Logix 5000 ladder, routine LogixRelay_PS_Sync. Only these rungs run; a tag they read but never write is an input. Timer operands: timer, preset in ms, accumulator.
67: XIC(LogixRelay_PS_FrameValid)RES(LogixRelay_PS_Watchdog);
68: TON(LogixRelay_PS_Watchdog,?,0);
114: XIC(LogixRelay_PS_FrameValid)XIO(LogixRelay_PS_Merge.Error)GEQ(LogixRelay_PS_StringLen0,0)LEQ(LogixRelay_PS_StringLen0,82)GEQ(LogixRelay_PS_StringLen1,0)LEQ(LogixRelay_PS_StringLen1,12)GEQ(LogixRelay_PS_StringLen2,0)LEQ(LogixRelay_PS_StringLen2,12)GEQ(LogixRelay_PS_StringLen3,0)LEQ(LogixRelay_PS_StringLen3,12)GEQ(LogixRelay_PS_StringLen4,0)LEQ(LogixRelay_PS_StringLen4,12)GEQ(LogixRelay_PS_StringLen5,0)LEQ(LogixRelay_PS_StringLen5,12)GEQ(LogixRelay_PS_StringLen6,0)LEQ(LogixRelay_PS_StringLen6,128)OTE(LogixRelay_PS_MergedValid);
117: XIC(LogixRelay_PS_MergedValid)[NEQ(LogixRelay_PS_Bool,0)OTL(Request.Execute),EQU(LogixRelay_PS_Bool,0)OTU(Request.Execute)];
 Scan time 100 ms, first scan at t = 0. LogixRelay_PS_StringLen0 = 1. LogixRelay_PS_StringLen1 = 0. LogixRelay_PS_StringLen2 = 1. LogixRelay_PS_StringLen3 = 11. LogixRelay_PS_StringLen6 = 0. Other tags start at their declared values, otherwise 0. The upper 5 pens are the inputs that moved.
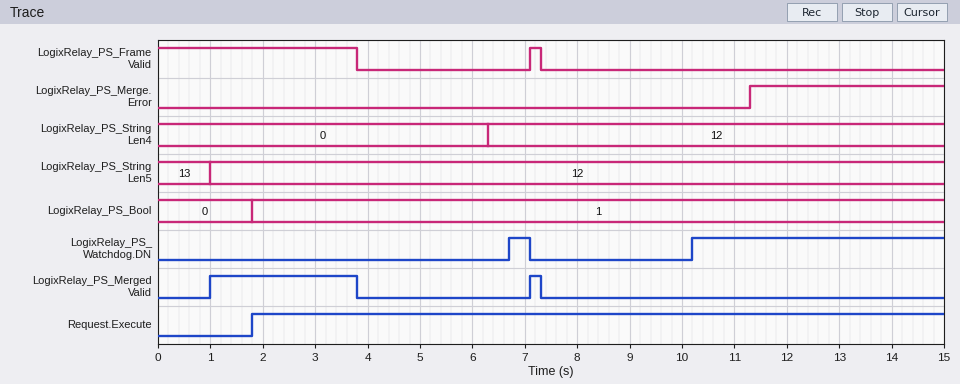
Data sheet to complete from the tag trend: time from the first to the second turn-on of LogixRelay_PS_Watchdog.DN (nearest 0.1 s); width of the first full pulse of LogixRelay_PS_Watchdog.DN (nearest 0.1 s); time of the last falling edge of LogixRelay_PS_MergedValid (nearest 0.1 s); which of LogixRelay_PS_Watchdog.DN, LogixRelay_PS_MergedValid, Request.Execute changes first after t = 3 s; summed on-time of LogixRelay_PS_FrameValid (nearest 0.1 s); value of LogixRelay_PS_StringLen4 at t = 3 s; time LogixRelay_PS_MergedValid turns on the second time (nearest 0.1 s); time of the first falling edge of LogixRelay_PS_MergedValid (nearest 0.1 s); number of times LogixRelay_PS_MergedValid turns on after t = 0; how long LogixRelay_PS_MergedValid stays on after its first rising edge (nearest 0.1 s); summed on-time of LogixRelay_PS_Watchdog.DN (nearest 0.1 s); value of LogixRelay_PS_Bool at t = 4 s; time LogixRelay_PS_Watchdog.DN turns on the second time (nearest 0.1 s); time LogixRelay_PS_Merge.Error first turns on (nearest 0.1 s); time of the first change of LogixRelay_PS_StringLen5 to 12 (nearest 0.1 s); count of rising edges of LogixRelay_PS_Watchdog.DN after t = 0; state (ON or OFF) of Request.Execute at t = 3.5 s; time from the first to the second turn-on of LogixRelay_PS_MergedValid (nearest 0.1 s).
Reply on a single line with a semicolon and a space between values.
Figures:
3.5 s; 0.4 s; 7.3 s; LogixRelay_PS_MergedValid; 4.0 s; 0; 7.1 s; 3.8 s; 2; 2.8 s; 5.2 s; 1; 10.2 s; 11.3 s; 1.0 s; 2; ON; 6.1 s
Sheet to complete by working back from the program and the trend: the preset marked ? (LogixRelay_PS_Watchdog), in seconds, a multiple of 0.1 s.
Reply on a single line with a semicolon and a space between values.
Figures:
3.0 s
